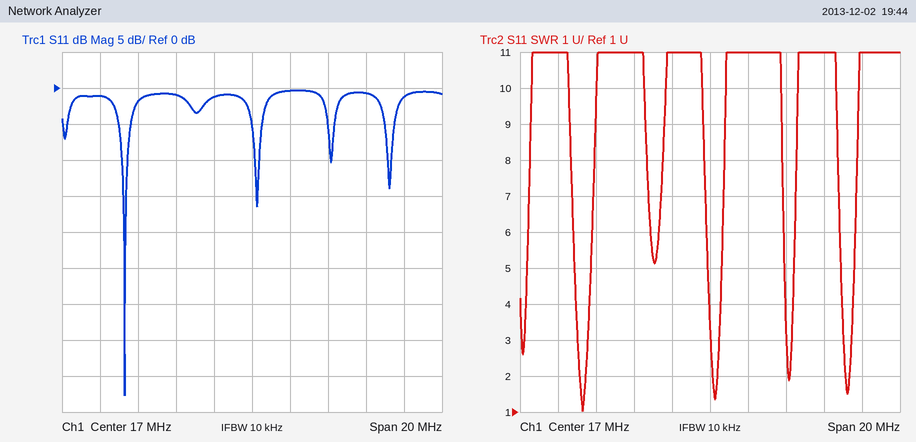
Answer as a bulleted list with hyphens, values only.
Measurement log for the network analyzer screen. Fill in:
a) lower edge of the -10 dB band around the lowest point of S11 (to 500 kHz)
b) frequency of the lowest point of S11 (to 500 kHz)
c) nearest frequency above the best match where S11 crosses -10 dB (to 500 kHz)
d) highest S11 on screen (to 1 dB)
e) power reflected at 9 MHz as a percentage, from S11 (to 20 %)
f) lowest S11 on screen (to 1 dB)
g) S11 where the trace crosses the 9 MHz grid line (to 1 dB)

- 10.0 MHz
- 10.5 MHz
- 10.5 MHz
- 0 dB
- 80 %
- -43 dB
- -1 dB
